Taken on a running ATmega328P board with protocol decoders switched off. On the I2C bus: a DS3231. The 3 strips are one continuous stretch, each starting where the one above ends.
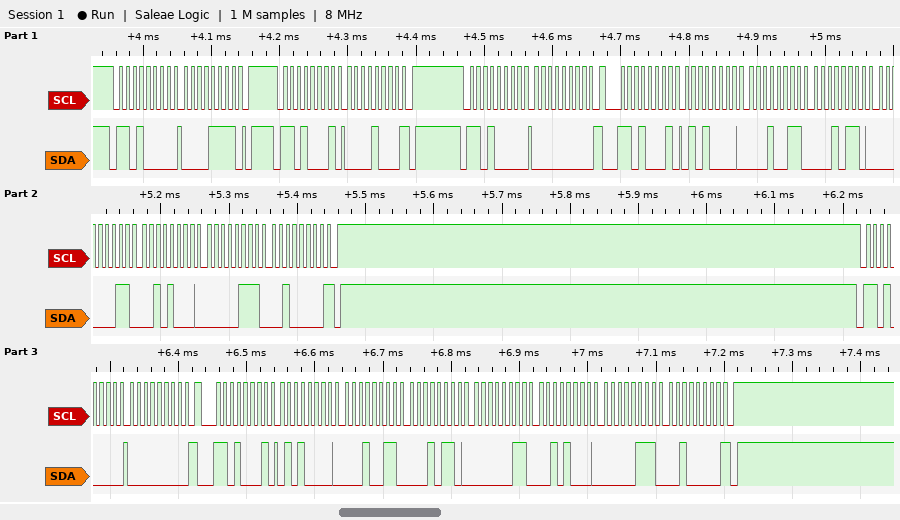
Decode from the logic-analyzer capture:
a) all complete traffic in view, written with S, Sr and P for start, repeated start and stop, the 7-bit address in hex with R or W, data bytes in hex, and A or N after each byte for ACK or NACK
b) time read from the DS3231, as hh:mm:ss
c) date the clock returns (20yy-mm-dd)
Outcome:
S 68W A 0F A P S 68R A 08 N P S 68W A 00 A Sr 68R A 50 A 13 A 16 A 03 A 28 A 07 A 20 N P S 68W A 00 A Sr 68R A 50 A 13 A 16 A 03 A 28 A 07 A 20 N P
16:13:50
2020-07-28
